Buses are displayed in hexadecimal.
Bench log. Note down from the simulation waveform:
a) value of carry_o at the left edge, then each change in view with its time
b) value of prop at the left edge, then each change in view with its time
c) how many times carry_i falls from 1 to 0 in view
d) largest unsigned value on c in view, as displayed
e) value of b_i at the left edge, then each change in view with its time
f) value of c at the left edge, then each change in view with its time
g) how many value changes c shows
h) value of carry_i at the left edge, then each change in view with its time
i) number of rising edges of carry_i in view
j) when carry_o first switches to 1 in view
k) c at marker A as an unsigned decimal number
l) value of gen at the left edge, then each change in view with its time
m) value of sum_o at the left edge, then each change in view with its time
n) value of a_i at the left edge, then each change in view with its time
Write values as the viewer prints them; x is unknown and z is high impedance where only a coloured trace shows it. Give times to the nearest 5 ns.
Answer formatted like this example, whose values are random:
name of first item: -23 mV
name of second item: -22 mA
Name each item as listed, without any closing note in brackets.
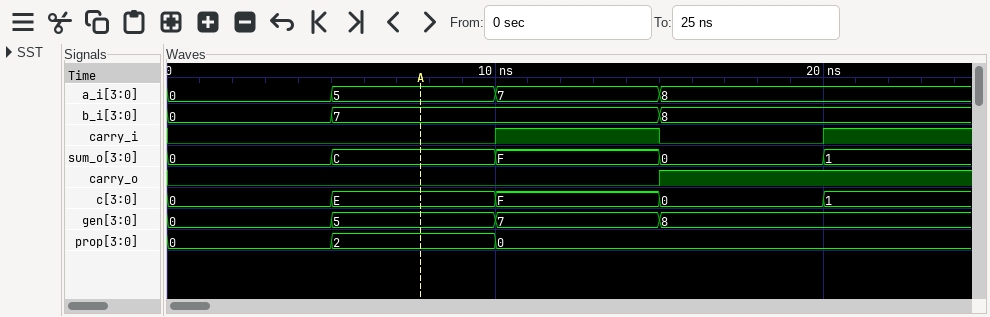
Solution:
value of carry_o at the left edge, then each change in view with its time: 0, 1 at 15 ns
value of prop at the left edge, then each change in view with its time: 0, 2 at 5 ns, 0 at 10 ns
how many times carry_i falls from 1 to 0 in view: 1
largest unsigned value on c in view, as displayed: F
value of b_i at the left edge, then each change in view with its time: 0, 7 at 5 ns, 8 at 15 ns
value of c at the left edge, then each change in view with its time: 0, E at 5 ns, F at 10 ns, 0 at 15 ns, 1 at 20 ns
how many value changes c shows: 4
value of carry_i at the left edge, then each change in view with its time: 0, 1 at 10 ns, 0 at 15 ns, 1 at 20 ns
number of rising edges of carry_i in view: 2
when carry_o first switches to 1 in view: 15 ns
c at marker A as an unsigned decimal number: 14
value of gen at the left edge, then each change in view with its time: 0, 5 at 5 ns, 7 at 10 ns, 8 at 15 ns
value of sum_o at the left edge, then each change in view with its time: 0, C at 5 ns, F at 10 ns, 0 at 15 ns, 1 at 20 ns
value of a_i at the left edge, then each change in view with its time: 0, 5 at 5 ns, 7 at 10 ns, 8 at 15 ns
